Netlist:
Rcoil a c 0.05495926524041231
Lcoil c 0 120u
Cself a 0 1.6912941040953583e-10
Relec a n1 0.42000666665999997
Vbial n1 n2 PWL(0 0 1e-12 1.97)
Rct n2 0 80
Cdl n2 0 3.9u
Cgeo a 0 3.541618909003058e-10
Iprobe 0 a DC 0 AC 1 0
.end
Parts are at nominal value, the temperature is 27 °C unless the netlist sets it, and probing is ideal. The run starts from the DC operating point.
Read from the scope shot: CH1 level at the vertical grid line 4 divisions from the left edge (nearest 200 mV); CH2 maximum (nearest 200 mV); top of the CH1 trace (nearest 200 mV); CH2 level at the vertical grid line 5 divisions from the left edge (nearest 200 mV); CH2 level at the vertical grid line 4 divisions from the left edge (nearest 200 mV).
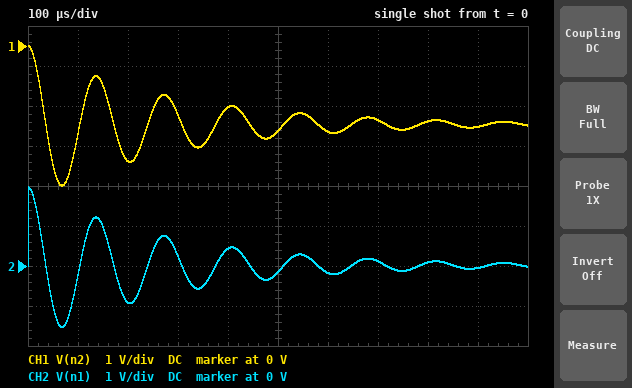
-1.6 V
2.0 V
0 V
-200 mV
400 mV
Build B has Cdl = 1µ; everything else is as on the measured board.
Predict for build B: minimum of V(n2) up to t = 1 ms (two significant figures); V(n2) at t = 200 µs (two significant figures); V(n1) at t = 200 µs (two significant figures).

-3.4 V
-1.7 V
300 mV
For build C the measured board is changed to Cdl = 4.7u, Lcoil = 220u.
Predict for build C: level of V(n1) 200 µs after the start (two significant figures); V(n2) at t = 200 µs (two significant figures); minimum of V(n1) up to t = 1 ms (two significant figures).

1.2 V
-760 mV
-1.5 V
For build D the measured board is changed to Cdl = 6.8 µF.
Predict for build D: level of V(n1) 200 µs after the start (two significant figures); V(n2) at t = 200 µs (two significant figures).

900 mV
-1.1 V
